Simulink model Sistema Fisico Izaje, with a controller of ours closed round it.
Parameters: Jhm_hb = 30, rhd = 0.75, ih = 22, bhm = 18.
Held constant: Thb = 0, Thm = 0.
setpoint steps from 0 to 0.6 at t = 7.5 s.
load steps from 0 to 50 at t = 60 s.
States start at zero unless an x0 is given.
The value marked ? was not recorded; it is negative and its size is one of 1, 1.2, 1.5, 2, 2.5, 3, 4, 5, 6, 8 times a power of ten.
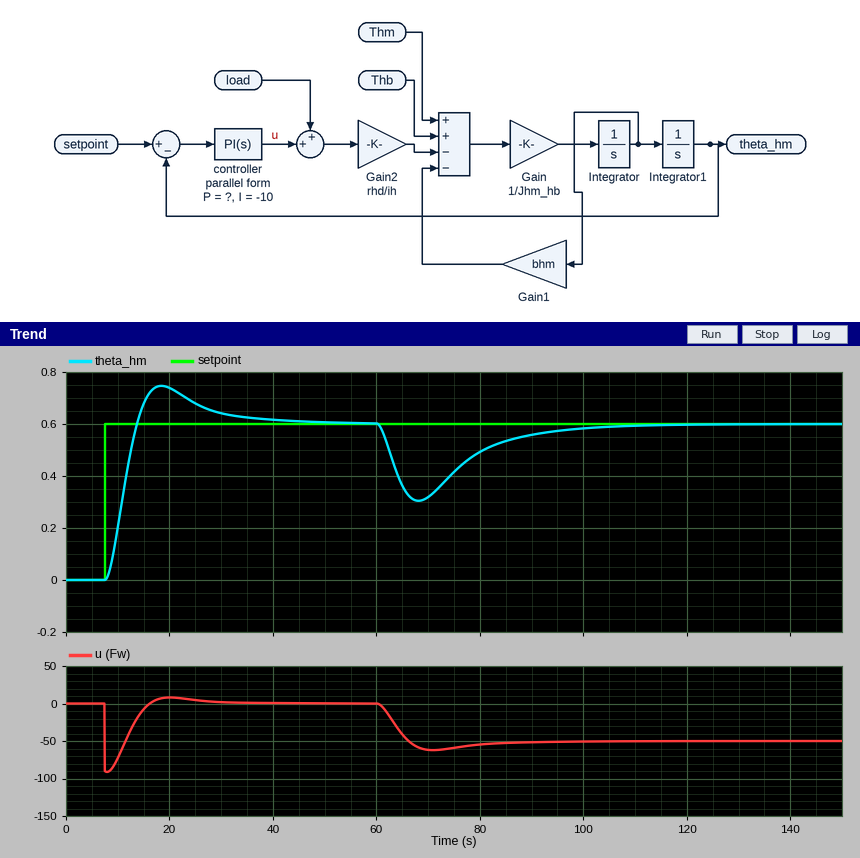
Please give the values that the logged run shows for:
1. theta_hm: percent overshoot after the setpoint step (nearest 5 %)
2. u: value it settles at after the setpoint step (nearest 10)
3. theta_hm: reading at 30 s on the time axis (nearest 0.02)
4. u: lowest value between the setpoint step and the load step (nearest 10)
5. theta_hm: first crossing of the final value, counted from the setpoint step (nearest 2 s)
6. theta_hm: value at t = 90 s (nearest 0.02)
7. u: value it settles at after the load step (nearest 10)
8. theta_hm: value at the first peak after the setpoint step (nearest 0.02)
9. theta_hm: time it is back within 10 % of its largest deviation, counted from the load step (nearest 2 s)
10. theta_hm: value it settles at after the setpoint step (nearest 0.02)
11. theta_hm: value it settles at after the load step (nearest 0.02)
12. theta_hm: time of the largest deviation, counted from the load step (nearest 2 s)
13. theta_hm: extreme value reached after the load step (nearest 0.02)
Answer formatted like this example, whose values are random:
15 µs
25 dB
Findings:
25 %
0
0.64
-90
6 s
0.56
-50
0.74
34 s
0.60
0.60
8 s
0.30
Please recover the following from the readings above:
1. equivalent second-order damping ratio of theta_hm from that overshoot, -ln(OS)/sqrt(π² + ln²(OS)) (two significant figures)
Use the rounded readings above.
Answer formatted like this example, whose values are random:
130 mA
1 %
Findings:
0.40
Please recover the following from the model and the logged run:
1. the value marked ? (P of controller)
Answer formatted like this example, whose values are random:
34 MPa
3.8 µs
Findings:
-150
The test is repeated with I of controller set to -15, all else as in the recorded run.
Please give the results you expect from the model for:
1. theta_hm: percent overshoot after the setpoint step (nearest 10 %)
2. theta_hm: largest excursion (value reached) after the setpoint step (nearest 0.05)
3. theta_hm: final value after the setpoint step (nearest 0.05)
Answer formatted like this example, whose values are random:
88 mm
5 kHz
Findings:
30 %
0.80
0.60
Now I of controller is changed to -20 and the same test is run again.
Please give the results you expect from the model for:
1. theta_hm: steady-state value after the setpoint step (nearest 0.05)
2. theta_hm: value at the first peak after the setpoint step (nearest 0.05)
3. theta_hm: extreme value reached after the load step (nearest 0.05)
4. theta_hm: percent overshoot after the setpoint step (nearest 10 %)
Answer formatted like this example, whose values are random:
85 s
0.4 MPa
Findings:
0.60
0.85
0.35
40 %
